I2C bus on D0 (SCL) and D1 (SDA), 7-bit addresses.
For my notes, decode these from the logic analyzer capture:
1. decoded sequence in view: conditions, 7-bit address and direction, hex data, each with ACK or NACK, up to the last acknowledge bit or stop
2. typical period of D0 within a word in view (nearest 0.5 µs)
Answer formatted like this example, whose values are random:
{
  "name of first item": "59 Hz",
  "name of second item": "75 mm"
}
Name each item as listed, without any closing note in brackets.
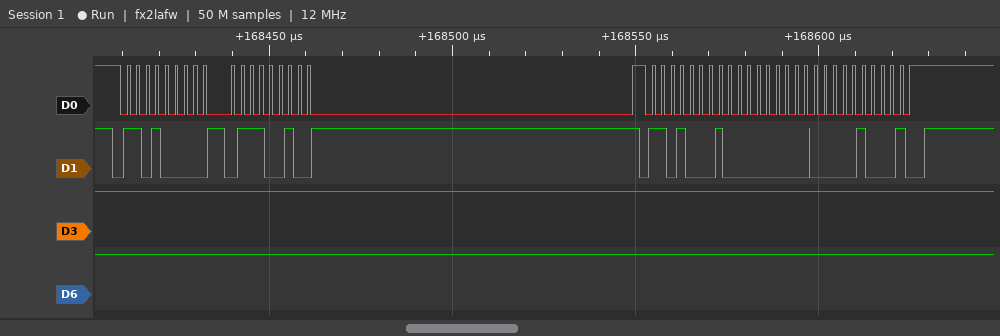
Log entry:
{
  "decoded sequence in view: conditions, 7-bit address and direction, hex data, each with ACK or NACK, up to the last acknowledge bit or stop": "start, address 68 write ACK, 72 ACK, repeated start, address 68 read ACK, 00 ACK, 08 NACK, stop",
  "typical period of D0 within a word in view": "2.5 µs"
}
